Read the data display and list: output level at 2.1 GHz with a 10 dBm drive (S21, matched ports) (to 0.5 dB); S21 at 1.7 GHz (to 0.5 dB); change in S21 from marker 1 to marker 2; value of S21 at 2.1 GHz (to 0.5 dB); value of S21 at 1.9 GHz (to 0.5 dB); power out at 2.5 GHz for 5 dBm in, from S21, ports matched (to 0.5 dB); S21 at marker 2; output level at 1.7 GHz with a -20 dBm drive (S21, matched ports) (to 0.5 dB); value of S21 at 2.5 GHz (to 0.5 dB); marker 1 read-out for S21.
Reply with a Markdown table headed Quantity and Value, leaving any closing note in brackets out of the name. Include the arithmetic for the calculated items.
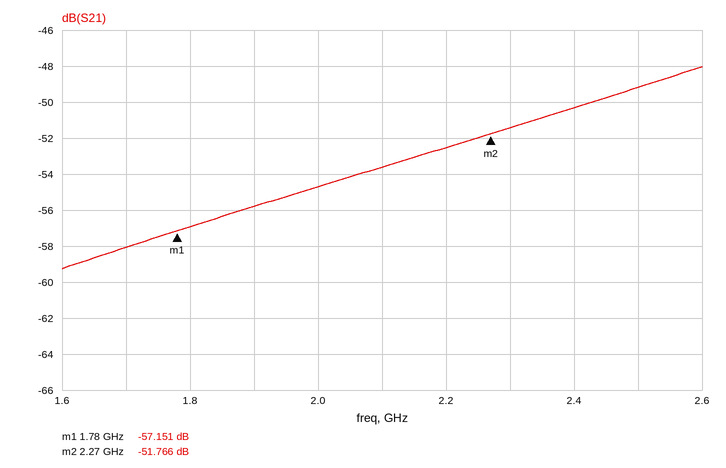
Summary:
| Quantity | Value |
|---|---|
| output level at 2.1 GHz with a 10 dBm drive (S21, matched ports) | 10 dBm + (-53.5 dB) = -43.5 dBm |
| S21 at 1.7 GHz | -58.0 dB |
| change in S21 from marker 1 to marker 2 | -51.766 − (-57.151) = 5.385 dB |
| value of S21 at 2.1 GHz | -53.5 dB |
| value of S21 at 1.9 GHz | -56.0 dB |
| power out at 2.5 GHz for 5 dBm in, from S21, ports matched | 5 dBm + (-49.0 dB) = -44.0 dBm |
| S21 at marker 2 | -51.766 dB |
| output level at 1.7 GHz with a -20 dBm drive (S21, matched ports) | -20 dBm + (-58.0 dB) = -78.0 dBm |
| value of S21 at 2.5 GHz | -49.0 dB |
| marker 1 read-out for S21 | -57.151 dB |
